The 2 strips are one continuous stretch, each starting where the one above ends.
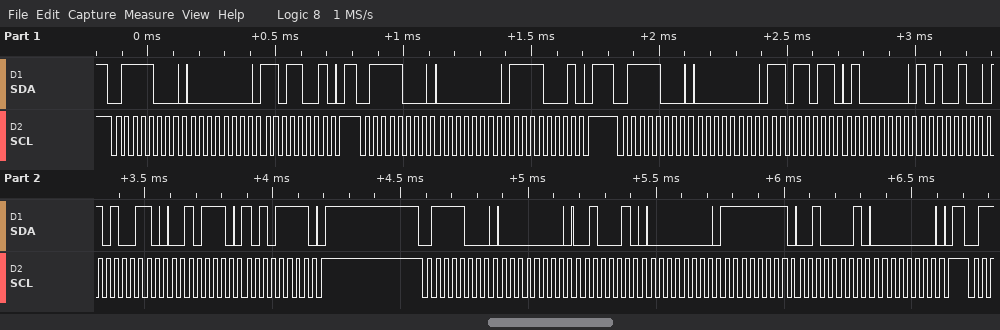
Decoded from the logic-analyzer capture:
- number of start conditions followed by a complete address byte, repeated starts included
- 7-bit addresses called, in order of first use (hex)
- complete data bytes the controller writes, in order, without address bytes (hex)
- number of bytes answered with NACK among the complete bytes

4
0x3C
00 D9 00 F1 00 DB 40 A4 A6 2E AF 00 22 00 FF 21 00
0
